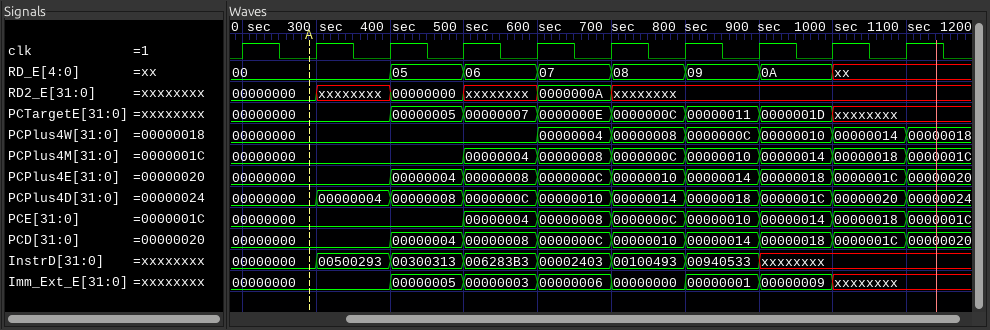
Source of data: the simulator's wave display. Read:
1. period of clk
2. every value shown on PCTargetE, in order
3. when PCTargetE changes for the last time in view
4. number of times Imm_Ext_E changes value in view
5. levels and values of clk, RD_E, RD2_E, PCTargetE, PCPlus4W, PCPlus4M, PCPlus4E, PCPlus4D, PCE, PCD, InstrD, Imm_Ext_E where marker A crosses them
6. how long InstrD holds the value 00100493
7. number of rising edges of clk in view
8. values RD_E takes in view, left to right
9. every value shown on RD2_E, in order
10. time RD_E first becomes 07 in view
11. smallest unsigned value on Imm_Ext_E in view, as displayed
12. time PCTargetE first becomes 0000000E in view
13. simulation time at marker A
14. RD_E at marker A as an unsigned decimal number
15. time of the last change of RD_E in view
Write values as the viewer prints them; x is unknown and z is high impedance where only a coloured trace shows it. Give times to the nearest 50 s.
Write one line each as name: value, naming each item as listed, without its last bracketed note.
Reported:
period of clk: 100 s
every value shown on PCTargetE, in order: 00000000, 00000005, 00000007, 0000000E, 0000000C, 00000011, 0000001D, xxxxxxxx
when PCTargetE changes for the last time in view: 1000 s
number of times Imm_Ext_E changes value in view: 7
levels and values of clk, RD_E, RD2_E, PCTargetE, PCPlus4W, PCPlus4M, PCPlus4E, PCPlus4D, PCE, PCD, InstrD, Imm_Ext_E where marker A crosses them: clk=0, RD_E=00, RD2_E=00000000, PCTargetE=00000000, PCPlus4W=00000000, PCPlus4M=00000000, PCPlus4E=00000000, PCPlus4D=00000000, PCE=00000000, PCD=00000000, InstrD=00000000, Imm_Ext_E=00000000
how long InstrD holds the value 00100493: 100 s
number of rising edges of clk in view: 10
values RD_E takes in view, left to right: 00, 05, 06, 07, 08, 09, 0A, xx
every value shown on RD2_E, in order: 00000000, xxxxxxxx, 00000000, xxxxxxxx, 0000000A, xxxxxxxx
time RD_E first becomes 07 in view: 600 s
smallest unsigned value on Imm_Ext_E in view, as displayed: 00000000
time PCTargetE first becomes 0000000E in view: 600 s
simulation time at marker A: 300 s
RD_E at marker A as an unsigned decimal number: 0
time of the last change of RD_E in view: 1000 s
